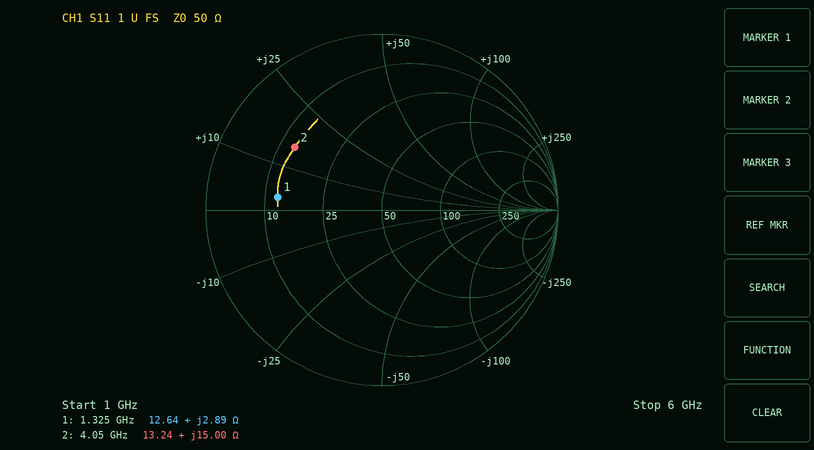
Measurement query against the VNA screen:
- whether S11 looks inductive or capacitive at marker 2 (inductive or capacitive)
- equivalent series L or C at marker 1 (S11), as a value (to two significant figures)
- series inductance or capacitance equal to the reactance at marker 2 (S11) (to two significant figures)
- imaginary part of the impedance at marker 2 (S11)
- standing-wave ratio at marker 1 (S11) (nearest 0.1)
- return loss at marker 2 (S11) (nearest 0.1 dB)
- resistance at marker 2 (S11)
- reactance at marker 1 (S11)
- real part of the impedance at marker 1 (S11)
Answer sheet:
inductive
350 pH
590 pH
+15.00 Ω
4.0
4.3 dB
13.24 Ω
+2.89 Ω
12.64 Ω
